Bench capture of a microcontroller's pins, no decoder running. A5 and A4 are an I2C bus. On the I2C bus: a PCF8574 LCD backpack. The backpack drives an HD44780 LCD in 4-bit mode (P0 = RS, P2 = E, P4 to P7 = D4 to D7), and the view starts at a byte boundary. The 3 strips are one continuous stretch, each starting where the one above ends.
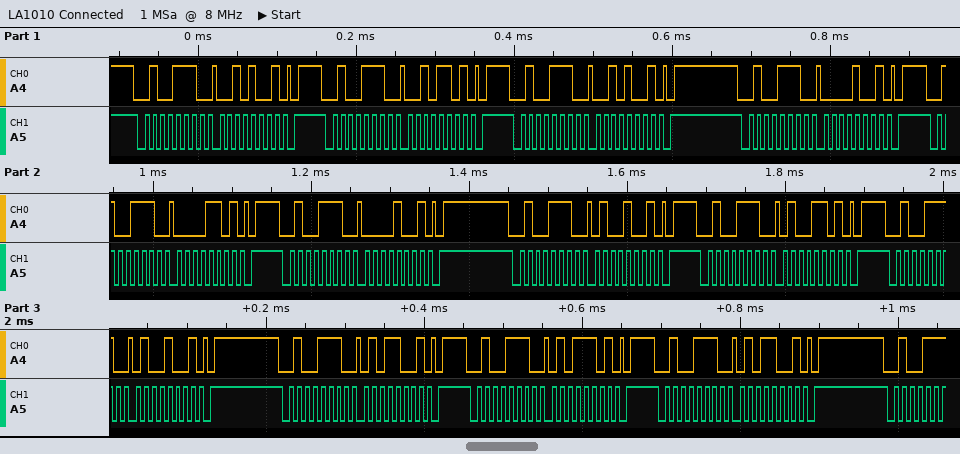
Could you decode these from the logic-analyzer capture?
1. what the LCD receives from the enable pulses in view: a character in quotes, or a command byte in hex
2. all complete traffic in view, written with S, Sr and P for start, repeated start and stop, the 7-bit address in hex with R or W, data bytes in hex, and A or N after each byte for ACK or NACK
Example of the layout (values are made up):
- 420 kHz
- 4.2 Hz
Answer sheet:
- ' ' 'E'
- S 27W A 29 A P S 27W A 2D A P S 27W A 29 A P S 27W A 09 A P S 27W A 0D A P S 27W A 09 A P S 27W A 49 A P S 27W A 4D A P S 27W A 49 A P S 27W A 59 A P S 27W A 5D A P S 27W A 59 A P
